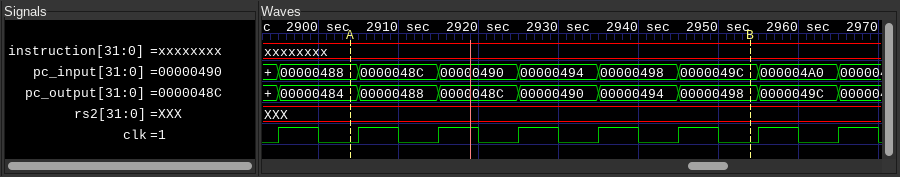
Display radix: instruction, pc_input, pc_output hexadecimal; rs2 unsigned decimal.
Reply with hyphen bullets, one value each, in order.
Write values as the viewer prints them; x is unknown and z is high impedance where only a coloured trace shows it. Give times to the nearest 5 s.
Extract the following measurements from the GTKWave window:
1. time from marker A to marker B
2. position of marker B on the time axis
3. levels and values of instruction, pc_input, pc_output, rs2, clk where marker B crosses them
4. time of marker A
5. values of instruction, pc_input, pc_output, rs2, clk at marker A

- 50 s
- 2955 s
- instruction=xxxxxxxx, pc_input=0000049C, pc_output=00000498, rs2=XXX, clk=0
- 2905 s
- instruction=xxxxxxxx, pc_input=00000488, pc_output=00000484, rs2=XXX, clk=0
